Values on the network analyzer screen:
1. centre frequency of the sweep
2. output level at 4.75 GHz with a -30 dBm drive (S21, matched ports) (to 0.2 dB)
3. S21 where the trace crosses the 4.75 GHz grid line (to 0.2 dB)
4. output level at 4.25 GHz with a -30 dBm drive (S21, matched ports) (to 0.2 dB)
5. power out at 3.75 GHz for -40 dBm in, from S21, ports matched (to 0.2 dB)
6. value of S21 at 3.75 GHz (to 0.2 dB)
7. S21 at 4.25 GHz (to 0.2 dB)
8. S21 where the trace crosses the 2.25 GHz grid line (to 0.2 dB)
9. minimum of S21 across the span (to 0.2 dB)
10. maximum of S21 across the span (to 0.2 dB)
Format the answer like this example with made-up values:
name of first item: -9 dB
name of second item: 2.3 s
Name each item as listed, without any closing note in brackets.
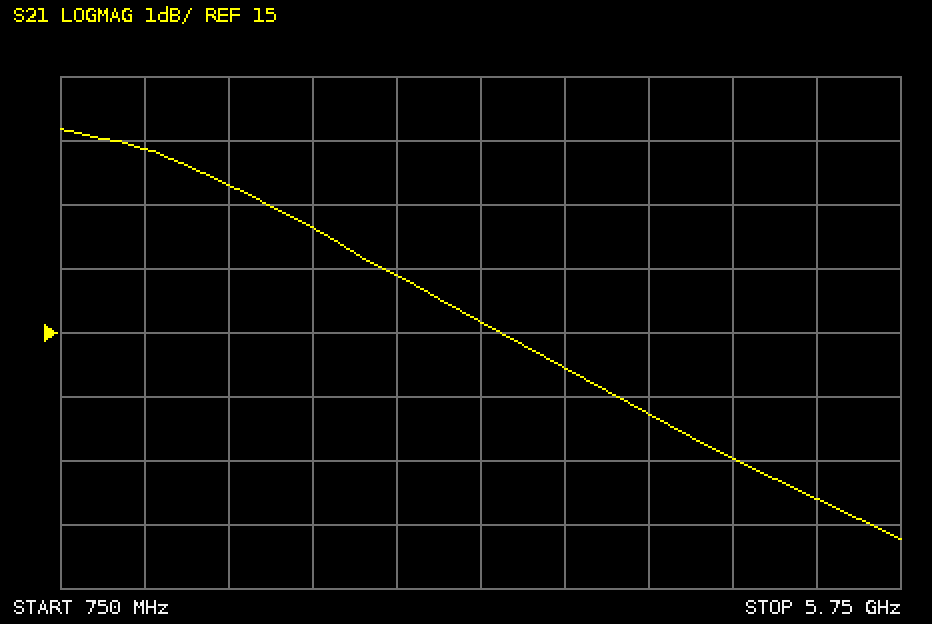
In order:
centre frequency of the sweep: 3.25 GHz
output level at 4.75 GHz with a -30 dBm drive (S21, matched ports): -17.0 dBm
S21 where the trace crosses the 4.75 GHz grid line: 13.0 dB
output level at 4.25 GHz with a -30 dBm drive (S21, matched ports): -16.2 dBm
power out at 3.75 GHz for -40 dBm in, from S21, ports matched: -25.6 dBm
value of S21 at 3.75 GHz: 14.4 dB
S21 at 4.25 GHz: 13.8 dB
S21 where the trace crosses the 2.25 GHz grid line: 16.6 dB
minimum of S21 across the span: 11.8 dB
maximum of S21 across the span: 18.2 dB
